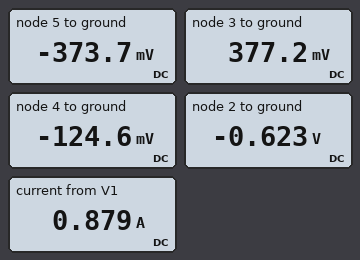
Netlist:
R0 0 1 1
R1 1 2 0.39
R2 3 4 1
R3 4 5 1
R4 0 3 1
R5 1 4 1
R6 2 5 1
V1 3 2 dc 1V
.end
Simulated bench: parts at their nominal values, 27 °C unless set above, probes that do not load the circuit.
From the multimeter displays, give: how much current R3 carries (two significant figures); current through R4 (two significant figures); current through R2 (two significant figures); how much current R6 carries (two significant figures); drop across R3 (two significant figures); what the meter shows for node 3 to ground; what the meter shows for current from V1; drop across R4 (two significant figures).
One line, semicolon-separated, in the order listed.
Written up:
250 mA; 380 mA; 500 mA; 250 mA; 250 mV; 377.2 mV; 0.879 A; 380 mV
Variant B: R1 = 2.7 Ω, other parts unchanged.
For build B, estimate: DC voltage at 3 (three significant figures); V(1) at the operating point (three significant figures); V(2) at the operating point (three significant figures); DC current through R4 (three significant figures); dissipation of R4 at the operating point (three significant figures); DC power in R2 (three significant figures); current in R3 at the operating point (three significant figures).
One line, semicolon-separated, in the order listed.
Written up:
194 mV; -194 mV; -806 mV; 194 mA; 37.6 mW; 126 mW; 322 mA
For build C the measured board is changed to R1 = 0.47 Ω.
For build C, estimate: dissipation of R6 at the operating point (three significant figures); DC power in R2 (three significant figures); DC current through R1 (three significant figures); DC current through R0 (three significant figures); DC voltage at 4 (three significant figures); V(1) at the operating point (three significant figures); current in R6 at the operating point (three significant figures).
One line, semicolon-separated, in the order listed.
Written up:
65.4 mW; 239 mW; 593 mA; 361 mA; -128 mV; -361 mV; 256 mA
